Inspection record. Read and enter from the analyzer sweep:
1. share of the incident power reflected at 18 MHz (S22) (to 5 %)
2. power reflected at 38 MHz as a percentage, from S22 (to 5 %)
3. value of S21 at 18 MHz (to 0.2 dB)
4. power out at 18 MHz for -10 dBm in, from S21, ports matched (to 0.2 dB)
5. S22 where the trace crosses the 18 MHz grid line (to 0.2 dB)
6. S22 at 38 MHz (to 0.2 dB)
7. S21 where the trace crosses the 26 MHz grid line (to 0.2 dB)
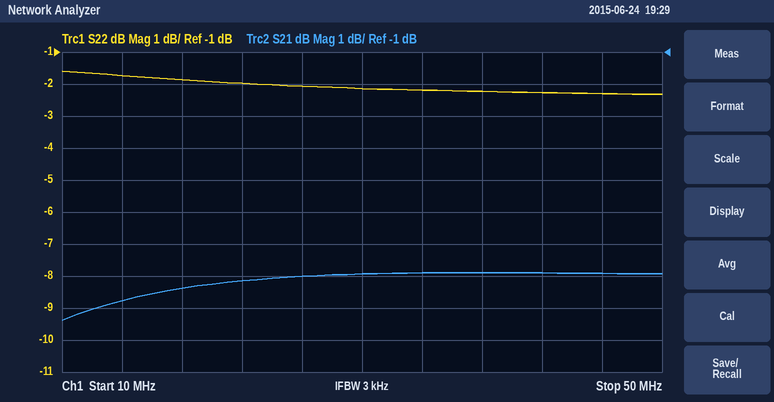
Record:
65 %
60 %
-8.4 dB
-18.4 dBm
-1.8 dB
-2.2 dB
-8.0 dB
